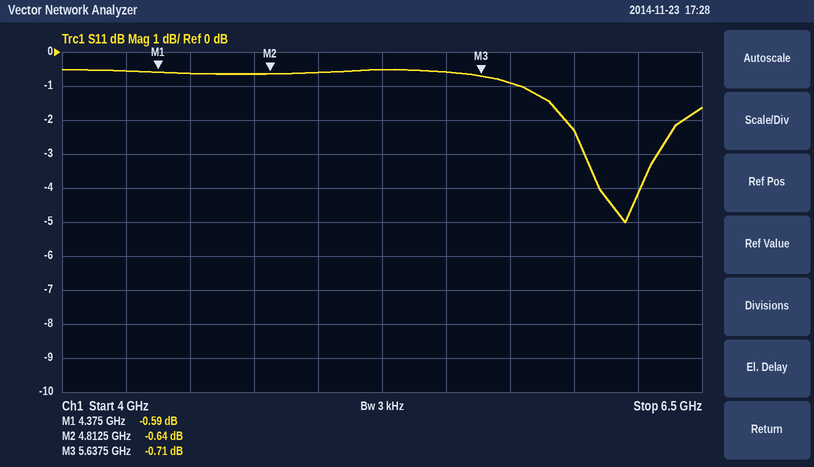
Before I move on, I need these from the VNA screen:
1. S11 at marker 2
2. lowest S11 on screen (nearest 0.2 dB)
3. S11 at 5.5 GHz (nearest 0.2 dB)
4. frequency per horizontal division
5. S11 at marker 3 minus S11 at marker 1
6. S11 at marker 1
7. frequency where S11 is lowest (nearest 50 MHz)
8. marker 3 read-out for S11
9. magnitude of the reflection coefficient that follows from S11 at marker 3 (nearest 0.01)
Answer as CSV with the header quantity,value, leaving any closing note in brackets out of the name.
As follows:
quantity,value
S11 at marker 2,-0.64 dB
lowest S11 on screen,-5.0 dB
S11 at 5.5 GHz,-0.6 dB
frequency per horizontal division,250 MHz
S11 at marker 3 minus S11 at marker 1,-0.12 dB
S11 at marker 1,-0.59 dB
frequency where S11 is lowest,6.20 GHz
marker 3 read-out for S11,-0.71 dB
magnitude of the reflection coefficient that follows from S11 at marker 3,0.92
